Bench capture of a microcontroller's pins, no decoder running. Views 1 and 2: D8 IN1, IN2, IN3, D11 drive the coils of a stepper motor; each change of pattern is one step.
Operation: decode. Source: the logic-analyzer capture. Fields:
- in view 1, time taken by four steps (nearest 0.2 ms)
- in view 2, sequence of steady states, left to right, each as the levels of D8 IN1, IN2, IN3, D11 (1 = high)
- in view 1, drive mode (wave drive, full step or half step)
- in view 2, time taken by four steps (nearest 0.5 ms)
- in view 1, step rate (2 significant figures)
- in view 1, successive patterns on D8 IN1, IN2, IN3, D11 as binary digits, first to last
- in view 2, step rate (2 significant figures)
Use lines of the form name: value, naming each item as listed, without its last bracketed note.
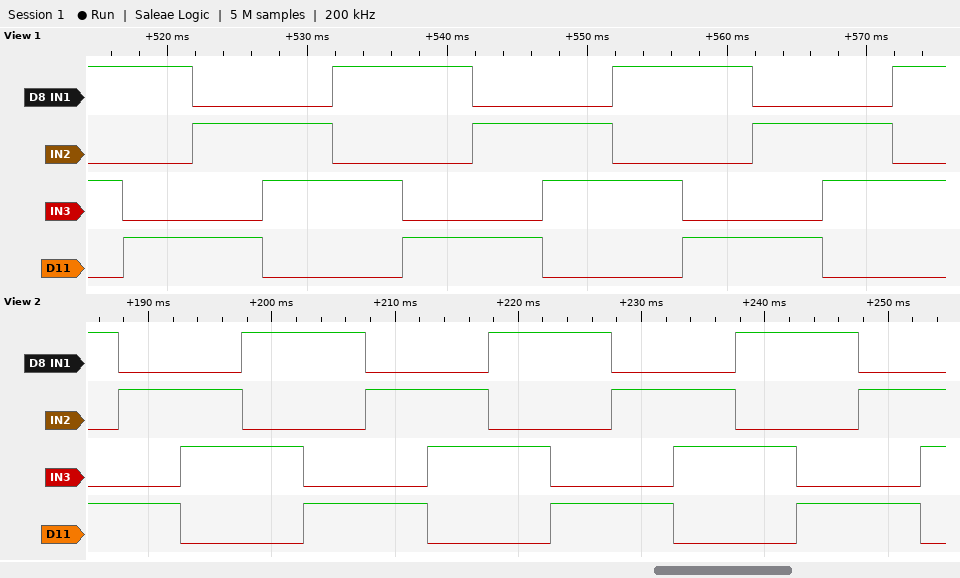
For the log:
in view 1, time taken by four steps: 20.0 ms
in view 2, sequence of steady states, left to right, each as the levels of D8 IN1, IN2, IN3, D11: 1001 0101 0110 1010 1001 0101 0110 1010 1001 0101 0110 1010 1001 0101 0110
in view 1, drive mode: full step
in view 2, time taken by four steps: 20.0 ms
in view 1, step rate: 200 steps/s
in view 1, successive patterns on D8 IN1, IN2, IN3, D11 as binary digits, first to last: 1010 1001 0101 0110 1010 1001 0101 0110 1010 1001 0101 0110 1010
in view 2, step rate: 200 steps/s
